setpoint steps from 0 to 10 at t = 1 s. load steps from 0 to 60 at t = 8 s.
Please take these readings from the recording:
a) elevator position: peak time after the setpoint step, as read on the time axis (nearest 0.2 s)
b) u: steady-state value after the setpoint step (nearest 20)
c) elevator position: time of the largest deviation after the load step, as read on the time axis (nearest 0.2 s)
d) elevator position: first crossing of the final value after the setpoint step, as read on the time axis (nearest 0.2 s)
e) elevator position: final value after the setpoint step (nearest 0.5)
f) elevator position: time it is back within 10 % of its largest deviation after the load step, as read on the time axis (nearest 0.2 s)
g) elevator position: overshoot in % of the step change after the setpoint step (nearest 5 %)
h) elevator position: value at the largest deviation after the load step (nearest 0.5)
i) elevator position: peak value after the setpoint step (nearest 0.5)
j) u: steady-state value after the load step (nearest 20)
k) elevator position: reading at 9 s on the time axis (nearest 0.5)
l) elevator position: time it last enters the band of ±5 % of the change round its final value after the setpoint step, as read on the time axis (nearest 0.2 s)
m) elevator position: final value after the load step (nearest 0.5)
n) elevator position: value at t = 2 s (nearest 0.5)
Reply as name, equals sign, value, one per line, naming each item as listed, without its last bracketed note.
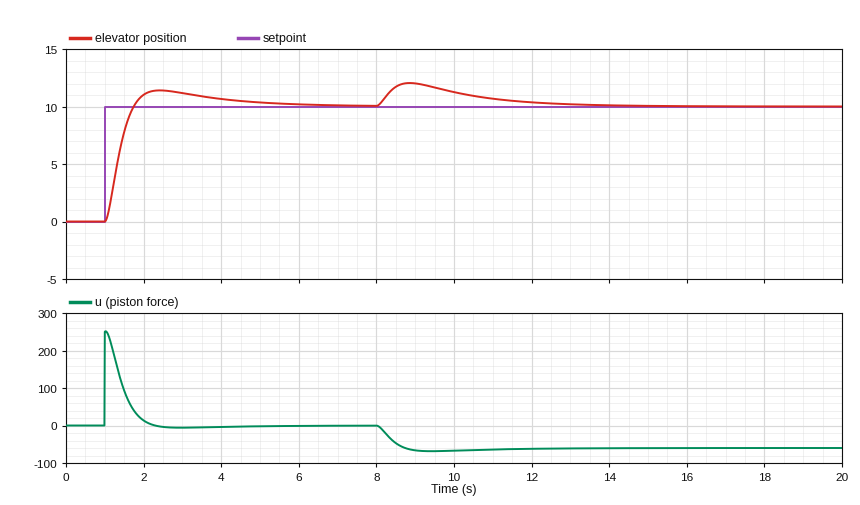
elevator position: peak time after the setpoint step, as read on the time axis = 2.4 s
u: steady-state value after the setpoint step = 0
elevator position: time of the largest deviation after the load step, as read on the time axis = 8.8 s
elevator position: first crossing of the final value after the setpoint step, as read on the time axis = 1.8 s
elevator position: final value after the setpoint step = 10.0
elevator position: time it is back within 10 % of its largest deviation after the load step, as read on the time axis = 13.0 s
elevator position: overshoot in % of the step change after the setpoint step = 15 %
elevator position: value at the largest deviation after the load step = 12.0
elevator position: peak value after the setpoint step = 11.5
u: steady-state value after the load step = -60
elevator position: reading at 9 s on the time axis = 12.0
elevator position: time it last enters the band of ±5 % of the change round its final value after the setpoint step, as read on the time axis = 4.4 s
elevator position: final value after the load step = 10.0
elevator position: value at t = 2 s = 11.0
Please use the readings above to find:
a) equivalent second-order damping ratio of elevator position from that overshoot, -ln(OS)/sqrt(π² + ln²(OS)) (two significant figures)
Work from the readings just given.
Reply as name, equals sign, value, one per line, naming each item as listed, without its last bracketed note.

equivalent second-order damping ratio of elevator position from that overshoot, -ln(OS)/sqrt(π² + ln²(OS)) = 0.52
